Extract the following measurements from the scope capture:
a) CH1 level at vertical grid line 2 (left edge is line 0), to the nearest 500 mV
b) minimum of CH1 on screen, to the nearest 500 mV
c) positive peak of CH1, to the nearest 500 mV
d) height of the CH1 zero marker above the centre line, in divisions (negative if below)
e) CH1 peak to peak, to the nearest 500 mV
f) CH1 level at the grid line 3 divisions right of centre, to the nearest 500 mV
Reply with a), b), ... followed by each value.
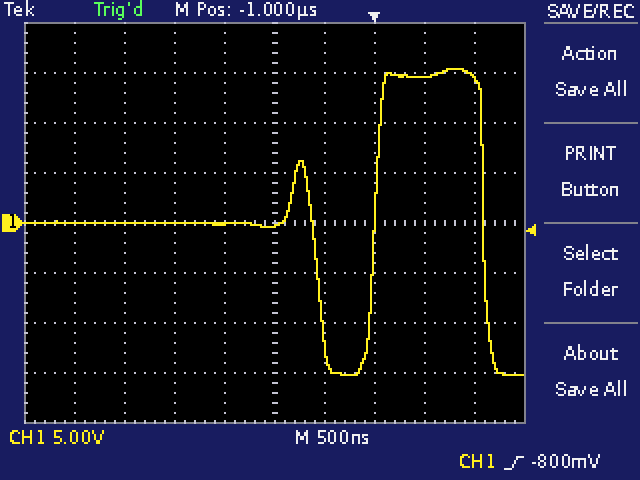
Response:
a) 0.0 V
b) -15.0 V
c) 15.5 V
d) 0.0 div
e) 30.5 V
f) 14.5 V
